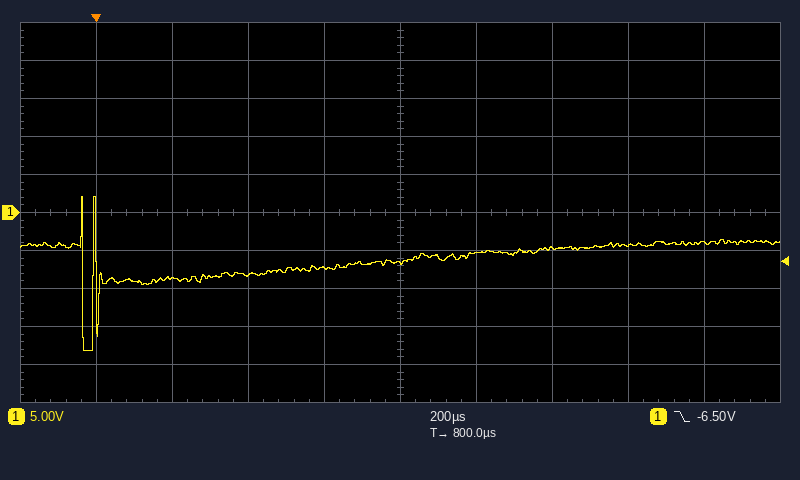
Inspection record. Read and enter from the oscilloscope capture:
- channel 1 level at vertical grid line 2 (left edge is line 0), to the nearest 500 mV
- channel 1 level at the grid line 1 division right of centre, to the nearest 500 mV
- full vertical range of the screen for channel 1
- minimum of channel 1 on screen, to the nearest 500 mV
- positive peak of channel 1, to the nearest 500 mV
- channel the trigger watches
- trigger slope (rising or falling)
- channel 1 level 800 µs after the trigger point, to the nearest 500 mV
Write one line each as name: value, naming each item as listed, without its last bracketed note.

channel 1 level at vertical grid line 2 (left edge is line 0), to the nearest 500 mV: -8.5 V
channel 1 level at the grid line 1 division right of centre, to the nearest 500 mV: -5.5 V
full vertical range of the screen for channel 1: 50 V
minimum of channel 1 on screen, to the nearest 500 mV: -18.0 V
positive peak of channel 1, to the nearest 500 mV: 2.0 V
channel the trigger watches: channel 1
trigger slope: falling
channel 1 level 800 µs after the trigger point, to the nearest 500 mV: -6.5 V
